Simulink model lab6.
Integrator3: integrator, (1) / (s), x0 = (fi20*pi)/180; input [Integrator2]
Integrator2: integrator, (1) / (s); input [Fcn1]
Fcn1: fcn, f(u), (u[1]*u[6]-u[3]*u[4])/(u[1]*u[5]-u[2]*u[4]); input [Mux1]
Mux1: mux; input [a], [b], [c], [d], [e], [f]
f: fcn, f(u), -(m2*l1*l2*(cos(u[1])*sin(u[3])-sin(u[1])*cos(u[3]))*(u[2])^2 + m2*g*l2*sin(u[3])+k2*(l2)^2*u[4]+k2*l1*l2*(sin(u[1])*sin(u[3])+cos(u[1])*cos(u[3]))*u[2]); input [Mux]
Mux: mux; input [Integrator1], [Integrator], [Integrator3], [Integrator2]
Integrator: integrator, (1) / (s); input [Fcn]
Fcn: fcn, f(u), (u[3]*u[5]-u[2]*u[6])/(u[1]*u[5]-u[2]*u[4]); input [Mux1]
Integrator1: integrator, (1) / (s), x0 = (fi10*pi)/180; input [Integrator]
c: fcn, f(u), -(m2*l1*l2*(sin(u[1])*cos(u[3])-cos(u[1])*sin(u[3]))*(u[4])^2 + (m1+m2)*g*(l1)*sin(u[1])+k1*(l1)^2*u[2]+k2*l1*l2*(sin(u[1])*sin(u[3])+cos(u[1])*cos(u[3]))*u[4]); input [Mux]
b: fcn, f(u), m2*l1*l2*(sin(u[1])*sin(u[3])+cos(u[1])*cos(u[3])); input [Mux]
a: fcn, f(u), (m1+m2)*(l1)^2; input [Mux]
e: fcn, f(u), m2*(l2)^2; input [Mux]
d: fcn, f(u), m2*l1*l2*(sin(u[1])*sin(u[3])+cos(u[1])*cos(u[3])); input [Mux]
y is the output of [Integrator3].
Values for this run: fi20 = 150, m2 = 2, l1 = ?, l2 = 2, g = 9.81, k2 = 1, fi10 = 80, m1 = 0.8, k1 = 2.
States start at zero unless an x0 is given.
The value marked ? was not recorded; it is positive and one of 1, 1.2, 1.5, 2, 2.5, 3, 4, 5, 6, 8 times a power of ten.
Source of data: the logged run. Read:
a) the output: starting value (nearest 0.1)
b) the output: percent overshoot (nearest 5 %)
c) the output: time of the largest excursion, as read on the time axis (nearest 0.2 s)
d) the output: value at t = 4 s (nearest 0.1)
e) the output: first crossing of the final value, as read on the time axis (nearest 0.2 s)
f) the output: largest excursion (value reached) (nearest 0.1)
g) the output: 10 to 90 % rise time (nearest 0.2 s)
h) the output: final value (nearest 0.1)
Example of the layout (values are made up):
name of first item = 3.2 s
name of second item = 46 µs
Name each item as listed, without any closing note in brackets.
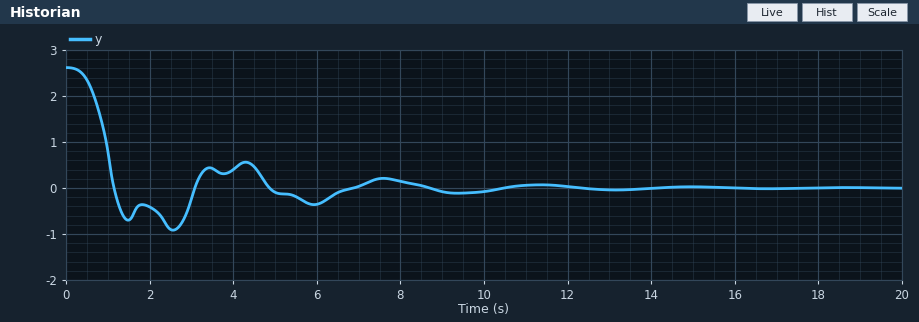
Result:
the output: starting value = 2.6
the output: percent overshoot = 35 %
the output: time of the largest excursion, as read on the time axis = 2.6 s
the output: value at t = 4 s = 0.4
the output: first crossing of the final value, as read on the time axis = 1.2 s
the output: largest excursion (value reached) = -0.9
the output: 10 to 90 % rise time = 0.6 s
the output: final value = 0.0
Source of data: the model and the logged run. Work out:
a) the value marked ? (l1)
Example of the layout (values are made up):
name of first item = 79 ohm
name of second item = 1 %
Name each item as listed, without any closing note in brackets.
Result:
the value marked ? = 1.5
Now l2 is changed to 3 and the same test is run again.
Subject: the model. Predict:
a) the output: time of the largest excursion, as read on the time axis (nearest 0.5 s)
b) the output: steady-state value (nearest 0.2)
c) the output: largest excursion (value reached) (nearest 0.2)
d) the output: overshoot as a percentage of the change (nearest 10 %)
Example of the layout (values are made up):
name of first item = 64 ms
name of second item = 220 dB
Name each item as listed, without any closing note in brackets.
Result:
the output: time of the largest excursion, as read on the time axis = 3.0 s
the output: steady-state value = 0.0
the output: largest excursion (value reached) = -0.8
the output: overshoot as a percentage of the change = 30 %
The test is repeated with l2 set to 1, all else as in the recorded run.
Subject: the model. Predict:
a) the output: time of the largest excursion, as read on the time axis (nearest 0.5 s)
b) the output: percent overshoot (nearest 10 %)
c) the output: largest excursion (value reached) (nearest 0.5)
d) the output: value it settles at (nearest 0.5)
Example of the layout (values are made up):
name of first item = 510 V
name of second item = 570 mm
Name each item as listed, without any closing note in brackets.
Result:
the output: time of the largest excursion, as read on the time axis = 2.0 s
the output: percent overshoot = 50 %
the output: largest excursion (value reached) = -1.5
the output: value it settles at = 0.0
